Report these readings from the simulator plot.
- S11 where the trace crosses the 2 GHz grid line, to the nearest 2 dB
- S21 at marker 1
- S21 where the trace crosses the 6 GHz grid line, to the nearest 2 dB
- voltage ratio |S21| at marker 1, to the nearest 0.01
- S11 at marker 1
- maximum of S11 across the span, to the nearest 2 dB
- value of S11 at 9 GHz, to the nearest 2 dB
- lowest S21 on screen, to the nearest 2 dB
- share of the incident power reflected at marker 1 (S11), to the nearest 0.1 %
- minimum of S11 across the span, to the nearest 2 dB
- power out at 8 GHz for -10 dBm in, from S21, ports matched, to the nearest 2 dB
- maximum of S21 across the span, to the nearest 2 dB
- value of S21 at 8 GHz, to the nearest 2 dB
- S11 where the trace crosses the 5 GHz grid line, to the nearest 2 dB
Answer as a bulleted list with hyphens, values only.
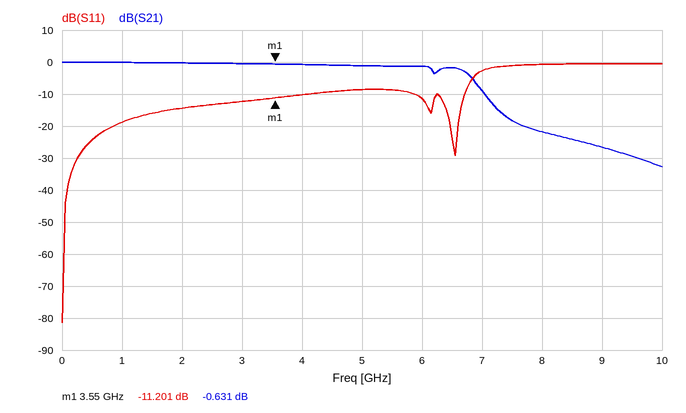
- -14 dB
- -0.631 dB
- -2 dB
- 0.93
- -11.201 dB
- 0 dB
- 0 dB
- -32 dB
- 7.6 %
- -82 dB
- -32 dBm
- 0 dB
- -22 dB
- -8 dB
